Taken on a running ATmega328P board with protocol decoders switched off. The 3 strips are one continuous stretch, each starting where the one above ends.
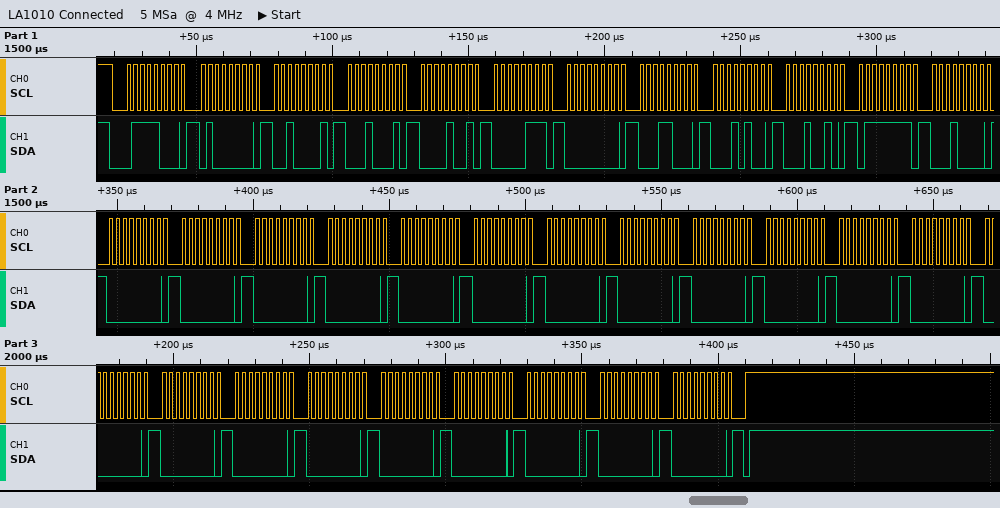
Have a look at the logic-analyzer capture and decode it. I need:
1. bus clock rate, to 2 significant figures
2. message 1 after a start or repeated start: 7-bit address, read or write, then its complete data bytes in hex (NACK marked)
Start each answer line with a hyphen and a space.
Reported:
- 400 kHz
- 0x3C write: 40 21 11 09 07 00 18 14 12 7F 10 00 00 00 00 00 00 00 00 00 00 00 00 00 00 00 00 00 00 00 00 00
